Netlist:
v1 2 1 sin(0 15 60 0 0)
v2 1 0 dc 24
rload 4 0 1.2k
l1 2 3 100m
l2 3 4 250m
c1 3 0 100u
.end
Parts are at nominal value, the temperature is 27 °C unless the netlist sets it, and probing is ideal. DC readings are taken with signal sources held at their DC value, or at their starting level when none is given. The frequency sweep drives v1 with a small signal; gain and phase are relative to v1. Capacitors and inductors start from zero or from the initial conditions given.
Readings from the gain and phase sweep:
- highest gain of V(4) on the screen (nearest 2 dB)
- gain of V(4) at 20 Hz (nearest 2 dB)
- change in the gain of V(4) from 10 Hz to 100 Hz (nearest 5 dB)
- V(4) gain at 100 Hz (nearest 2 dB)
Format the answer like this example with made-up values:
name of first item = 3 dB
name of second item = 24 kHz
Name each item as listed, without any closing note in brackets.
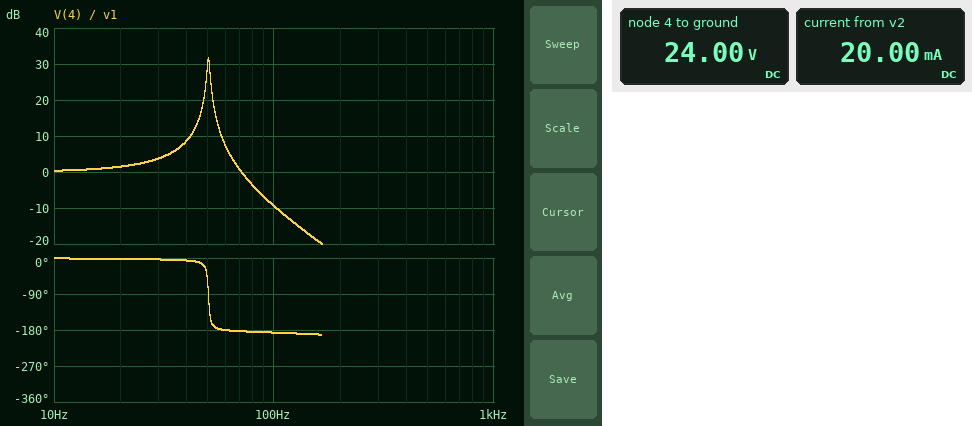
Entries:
highest gain of V(4) on the screen = 32 dB
gain of V(4) at 20 Hz = 2 dB
change in the gain of V(4) from 10 Hz to 100 Hz = -10 dB
V(4) gain at 100 Hz = -10 dB
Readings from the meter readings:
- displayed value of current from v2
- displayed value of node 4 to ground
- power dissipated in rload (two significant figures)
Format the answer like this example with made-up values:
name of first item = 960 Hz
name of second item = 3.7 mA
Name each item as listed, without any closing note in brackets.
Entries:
displayed value of current from v2 = 20.00 mA
displayed value of node 4 to ground = 24.00 V
power dissipated in rload = 480 mW
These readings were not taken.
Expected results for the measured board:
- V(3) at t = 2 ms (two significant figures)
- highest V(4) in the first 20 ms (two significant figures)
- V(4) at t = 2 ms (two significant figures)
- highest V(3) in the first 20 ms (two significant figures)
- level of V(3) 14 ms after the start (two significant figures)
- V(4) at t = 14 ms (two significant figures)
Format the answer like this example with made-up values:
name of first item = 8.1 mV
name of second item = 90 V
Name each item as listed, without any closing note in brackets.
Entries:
V(3) at t = 2 ms = 5.3 V
highest V(4) in the first 20 ms = 67 V
V(4) at t = 2 ms = 4.3 V
highest V(3) in the first 20 ms = 67 V
level of V(3) 14 ms after the start = 20 V
V(4) at t = 14 ms = 24 V
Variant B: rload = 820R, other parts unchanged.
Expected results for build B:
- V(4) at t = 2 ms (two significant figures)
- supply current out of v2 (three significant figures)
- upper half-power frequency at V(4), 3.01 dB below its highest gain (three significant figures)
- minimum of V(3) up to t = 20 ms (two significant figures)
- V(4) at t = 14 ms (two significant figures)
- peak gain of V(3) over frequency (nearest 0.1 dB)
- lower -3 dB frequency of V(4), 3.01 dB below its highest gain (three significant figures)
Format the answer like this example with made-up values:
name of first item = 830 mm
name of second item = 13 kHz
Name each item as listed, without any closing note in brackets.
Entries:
V(4) at t = 2 ms = 3.9 V
supply current out of v2 = 29.3 mA
upper half-power frequency at V(4), 3.01 dB below its highest gain = 51.4 Hz
minimum of V(3) up to t = 20 ms = -34 V
V(4) at t = 14 ms = 25 V
peak gain of V(3) over frequency = 28.3 dB
lower -3 dB frequency of V(4), 3.01 dB below its highest gain = 49.4 Hz
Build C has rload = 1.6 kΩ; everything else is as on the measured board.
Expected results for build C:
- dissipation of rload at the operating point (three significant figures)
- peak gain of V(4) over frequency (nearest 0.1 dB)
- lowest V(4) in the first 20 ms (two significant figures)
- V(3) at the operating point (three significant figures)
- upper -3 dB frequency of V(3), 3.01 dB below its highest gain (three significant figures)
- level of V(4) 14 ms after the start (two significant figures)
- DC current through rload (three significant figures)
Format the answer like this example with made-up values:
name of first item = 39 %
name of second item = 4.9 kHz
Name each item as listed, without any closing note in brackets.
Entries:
dissipation of rload at the operating point = 360 mW
peak gain of V(4) over frequency = 34.1 dB
lowest V(4) in the first 20 ms = -36 V
V(3) at the operating point = 24.0 V
upper -3 dB frequency of V(3), 3.01 dB below its highest gain = 50.8 Hz
level of V(4) 14 ms after the start = 23 V
DC current through rload = 15.0 mA
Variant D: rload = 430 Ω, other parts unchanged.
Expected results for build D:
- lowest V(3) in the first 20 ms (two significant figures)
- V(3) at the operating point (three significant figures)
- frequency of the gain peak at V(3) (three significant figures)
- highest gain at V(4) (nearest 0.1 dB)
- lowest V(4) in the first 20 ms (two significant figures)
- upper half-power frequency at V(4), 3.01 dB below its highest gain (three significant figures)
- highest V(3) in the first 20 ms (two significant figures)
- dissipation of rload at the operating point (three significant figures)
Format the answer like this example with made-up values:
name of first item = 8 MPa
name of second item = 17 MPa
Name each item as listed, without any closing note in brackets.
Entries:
lowest V(3) in the first 20 ms = -30 V
V(3) at the operating point = 24.0 V
frequency of the gain peak at V(3) = 50.6 Hz
highest gain at V(4) = 22.8 dB
lowest V(4) in the first 20 ms = -29 V
upper half-power frequency at V(4), 3.01 dB below its highest gain = 52.4 Hz
highest V(3) in the first 20 ms = 65 V
dissipation of rload at the operating point = 1.34 W
